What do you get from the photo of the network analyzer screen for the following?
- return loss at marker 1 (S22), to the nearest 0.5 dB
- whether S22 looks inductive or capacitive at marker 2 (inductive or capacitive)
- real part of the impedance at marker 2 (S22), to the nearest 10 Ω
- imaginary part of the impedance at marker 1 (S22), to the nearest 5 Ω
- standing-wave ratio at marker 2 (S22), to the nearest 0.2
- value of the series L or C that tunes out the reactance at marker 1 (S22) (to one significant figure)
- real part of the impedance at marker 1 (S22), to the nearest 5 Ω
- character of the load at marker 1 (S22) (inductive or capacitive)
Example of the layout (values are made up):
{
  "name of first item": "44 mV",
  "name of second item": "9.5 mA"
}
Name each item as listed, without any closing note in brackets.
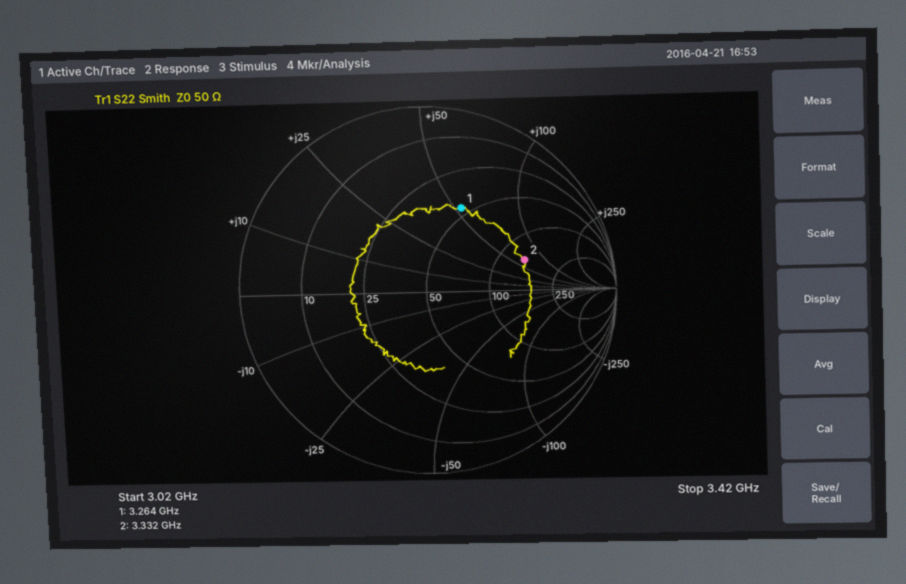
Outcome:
{
  "return loss at marker 1 (S22), to the nearest 0.5 dB": "6.0 dB",
  "whether S22 looks inductive or capacitive at marker 2": "inductive",
  "real part of the impedance at marker 2 (S22), to the nearest 10 Ω": "140 Ω",
  "imaginary part of the impedance at marker 1 (S22), to the nearest 5 Ω": "+55 Ω",
  "standing-wave ratio at marker 2 (S22), to the nearest 0.2": "3.4",
  "value of the series L or C that tunes out the reactance at marker 1 (S22)": "900 fF",
  "real part of the impedance at marker 1 (S22), to the nearest 5 Ω": "45 Ω",
  "character of the load at marker 1 (S22)": "inductive"
}
